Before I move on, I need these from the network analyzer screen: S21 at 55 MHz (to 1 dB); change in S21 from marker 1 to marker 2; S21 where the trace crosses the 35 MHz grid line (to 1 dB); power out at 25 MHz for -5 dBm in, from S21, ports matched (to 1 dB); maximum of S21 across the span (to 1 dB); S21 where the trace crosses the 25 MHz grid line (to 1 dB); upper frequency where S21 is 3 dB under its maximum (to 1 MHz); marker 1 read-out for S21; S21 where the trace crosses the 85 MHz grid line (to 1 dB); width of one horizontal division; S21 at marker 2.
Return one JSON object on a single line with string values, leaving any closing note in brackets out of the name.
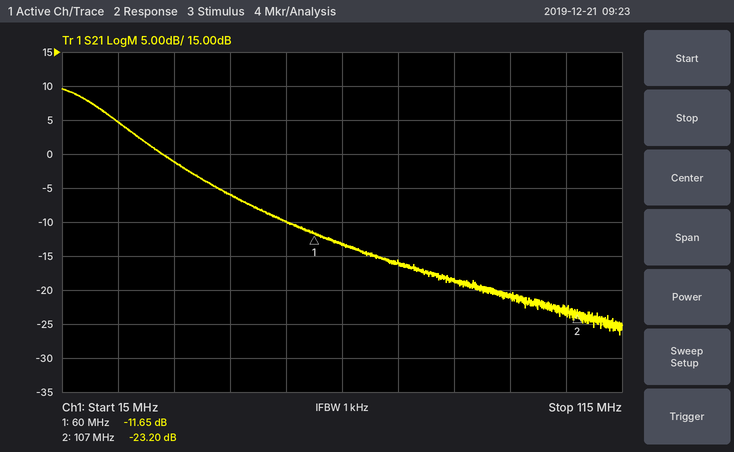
{"S21 at 55 MHz": "-10 dB", "change in S21 from marker 1 to marker 2": "-11.55 dB", "S21 where the trace crosses the 35 MHz grid line": "-1 dB", "power out at 25 MHz for -5 dBm in, from S21, ports matched": "0 dBm", "maximum of S21 across the span": "10 dB", "S21 where the trace crosses the 25 MHz grid line": "5 dB", "upper frequency where S21 is 3 dB under its maximum": "22 MHz", "marker 1 read-out for S21": "-11.65 dB", "S21 where the trace crosses the 85 MHz grid line": "-19 dB", "width of one horizontal division": "10 MHz", "S21 at marker 2": "-23.20 dB"}
